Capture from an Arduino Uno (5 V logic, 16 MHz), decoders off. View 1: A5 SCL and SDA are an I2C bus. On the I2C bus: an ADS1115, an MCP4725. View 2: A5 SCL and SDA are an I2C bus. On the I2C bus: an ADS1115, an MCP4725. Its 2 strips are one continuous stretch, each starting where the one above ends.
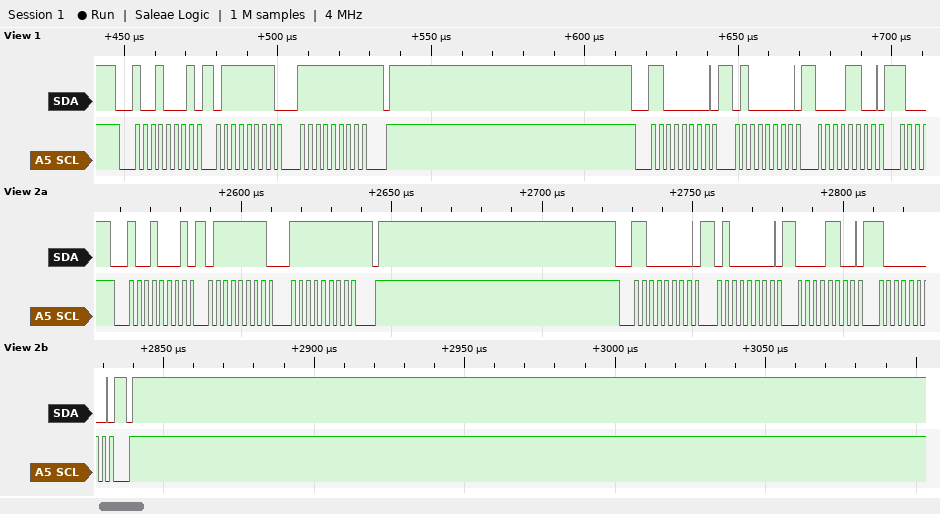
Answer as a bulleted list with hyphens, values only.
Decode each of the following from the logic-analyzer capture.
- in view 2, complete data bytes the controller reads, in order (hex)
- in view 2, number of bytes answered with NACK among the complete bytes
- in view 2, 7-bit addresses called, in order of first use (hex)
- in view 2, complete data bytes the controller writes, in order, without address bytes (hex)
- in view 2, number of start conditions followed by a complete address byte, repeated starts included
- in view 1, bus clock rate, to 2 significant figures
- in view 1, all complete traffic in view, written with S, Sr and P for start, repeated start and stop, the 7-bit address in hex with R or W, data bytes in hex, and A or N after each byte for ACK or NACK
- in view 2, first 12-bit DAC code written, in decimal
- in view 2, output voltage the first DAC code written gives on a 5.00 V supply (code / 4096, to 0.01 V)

- 7F FF
- 1
- 0x48 0x60
- 40 0C 80
- 2
- 400 kHz
- S 48R A 7F A FF N P S 60W A 40 A 0C A
- 200
- 0.24 V
